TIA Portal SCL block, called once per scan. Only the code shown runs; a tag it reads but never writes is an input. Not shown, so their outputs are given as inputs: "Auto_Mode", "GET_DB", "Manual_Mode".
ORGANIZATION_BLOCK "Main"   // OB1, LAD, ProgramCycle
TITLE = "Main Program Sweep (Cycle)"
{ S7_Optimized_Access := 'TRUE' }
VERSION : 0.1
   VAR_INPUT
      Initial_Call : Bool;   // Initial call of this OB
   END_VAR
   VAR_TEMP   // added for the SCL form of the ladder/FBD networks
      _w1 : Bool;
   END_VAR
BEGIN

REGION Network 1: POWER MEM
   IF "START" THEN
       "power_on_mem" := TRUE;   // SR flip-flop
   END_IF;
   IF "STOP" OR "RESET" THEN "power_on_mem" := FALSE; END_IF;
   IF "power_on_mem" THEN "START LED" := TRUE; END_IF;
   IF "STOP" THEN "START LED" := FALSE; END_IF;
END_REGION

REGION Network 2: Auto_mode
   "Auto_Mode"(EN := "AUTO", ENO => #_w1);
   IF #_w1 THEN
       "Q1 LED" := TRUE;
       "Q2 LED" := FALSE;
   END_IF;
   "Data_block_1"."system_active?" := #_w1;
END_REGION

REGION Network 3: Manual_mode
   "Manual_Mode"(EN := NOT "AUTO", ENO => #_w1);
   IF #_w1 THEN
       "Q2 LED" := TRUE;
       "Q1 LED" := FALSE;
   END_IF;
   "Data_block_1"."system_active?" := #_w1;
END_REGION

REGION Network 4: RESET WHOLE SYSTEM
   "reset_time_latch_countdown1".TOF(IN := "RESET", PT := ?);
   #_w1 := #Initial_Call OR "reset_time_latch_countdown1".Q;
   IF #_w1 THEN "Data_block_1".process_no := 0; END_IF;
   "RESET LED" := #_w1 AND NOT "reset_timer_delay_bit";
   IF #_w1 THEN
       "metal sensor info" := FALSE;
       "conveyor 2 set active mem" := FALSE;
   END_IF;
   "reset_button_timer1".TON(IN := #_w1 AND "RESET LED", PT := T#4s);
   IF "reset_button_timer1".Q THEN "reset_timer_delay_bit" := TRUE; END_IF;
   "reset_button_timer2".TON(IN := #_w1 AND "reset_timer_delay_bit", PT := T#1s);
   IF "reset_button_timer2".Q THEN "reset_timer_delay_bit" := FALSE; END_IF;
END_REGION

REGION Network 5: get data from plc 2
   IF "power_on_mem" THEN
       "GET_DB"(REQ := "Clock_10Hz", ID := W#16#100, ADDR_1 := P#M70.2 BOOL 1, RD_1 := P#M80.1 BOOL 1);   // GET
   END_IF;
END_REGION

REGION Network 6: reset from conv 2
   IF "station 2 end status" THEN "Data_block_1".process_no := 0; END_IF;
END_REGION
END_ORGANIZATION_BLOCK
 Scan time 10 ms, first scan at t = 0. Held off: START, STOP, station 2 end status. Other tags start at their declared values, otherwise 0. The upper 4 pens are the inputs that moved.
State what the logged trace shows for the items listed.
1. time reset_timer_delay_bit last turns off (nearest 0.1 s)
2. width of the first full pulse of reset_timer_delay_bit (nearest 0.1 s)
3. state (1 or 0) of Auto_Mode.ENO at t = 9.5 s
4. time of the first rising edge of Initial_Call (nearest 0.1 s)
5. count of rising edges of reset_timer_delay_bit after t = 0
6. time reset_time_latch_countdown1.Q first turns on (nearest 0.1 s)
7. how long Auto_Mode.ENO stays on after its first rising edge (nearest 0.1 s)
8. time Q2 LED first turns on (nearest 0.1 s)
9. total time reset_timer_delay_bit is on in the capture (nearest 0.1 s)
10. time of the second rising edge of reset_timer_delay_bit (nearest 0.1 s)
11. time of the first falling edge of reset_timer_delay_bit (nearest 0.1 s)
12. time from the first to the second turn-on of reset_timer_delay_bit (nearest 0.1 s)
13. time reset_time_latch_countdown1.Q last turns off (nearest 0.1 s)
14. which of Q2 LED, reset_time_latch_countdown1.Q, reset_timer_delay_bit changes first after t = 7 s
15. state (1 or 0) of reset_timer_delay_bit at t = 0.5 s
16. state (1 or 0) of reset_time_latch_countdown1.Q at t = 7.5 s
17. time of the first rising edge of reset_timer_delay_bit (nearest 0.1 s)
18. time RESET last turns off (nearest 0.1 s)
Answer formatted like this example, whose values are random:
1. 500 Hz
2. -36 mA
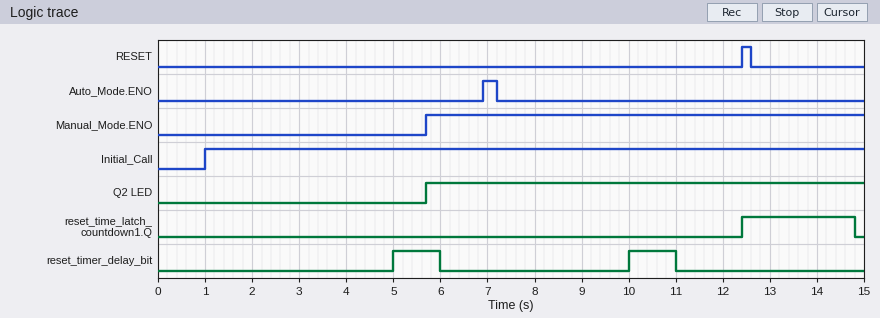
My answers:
1. 11.0 s
2. 1.0 s
3. 0
4. 1.0 s
5. 2
6. 12.4 s
7. 0.3 s
8. 5.7 s
9. 2.0 s
10. 10.0 s
11. 6.0 s
12. 5.0 s
13. 14.8 s
14. reset_timer_delay_bit
15. 0
16. 0
17. 5.0 s
18. 12.6 s
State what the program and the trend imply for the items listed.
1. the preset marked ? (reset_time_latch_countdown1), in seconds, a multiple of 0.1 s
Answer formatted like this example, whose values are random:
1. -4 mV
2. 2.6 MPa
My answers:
1. 2.2 s
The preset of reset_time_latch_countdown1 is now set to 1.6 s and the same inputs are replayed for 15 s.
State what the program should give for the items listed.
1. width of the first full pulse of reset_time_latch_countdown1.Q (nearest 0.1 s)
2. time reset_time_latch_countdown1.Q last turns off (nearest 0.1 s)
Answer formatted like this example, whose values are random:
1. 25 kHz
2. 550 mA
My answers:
1. 1.8 s
2. 14.2 s
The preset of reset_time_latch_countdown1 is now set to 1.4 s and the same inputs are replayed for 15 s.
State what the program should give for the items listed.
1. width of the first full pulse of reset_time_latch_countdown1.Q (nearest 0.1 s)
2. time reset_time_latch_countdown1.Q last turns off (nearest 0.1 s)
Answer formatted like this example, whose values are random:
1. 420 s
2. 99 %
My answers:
1. 1.6 s
2. 14.0 s
